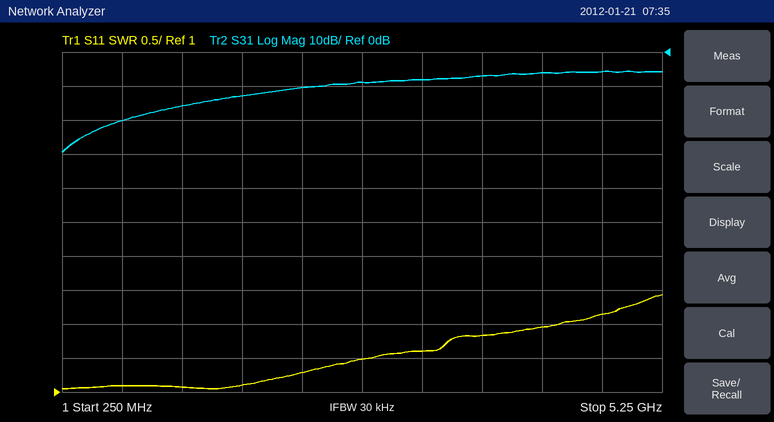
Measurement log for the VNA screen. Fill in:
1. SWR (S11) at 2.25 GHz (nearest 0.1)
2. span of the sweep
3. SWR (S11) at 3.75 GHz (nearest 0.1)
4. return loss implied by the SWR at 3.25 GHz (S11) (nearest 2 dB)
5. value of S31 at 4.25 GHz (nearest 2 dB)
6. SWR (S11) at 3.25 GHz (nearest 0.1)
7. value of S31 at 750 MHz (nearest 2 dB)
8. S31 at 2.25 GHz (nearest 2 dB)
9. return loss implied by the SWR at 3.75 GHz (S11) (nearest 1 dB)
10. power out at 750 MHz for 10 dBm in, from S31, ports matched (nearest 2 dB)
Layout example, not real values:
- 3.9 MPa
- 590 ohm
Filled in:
- 1.3
- 5 GHz
- 1.8
- 12 dB
- -6 dB
- 1.6
- -20 dB
- -10 dB
- 11 dB
- -10 dBm
